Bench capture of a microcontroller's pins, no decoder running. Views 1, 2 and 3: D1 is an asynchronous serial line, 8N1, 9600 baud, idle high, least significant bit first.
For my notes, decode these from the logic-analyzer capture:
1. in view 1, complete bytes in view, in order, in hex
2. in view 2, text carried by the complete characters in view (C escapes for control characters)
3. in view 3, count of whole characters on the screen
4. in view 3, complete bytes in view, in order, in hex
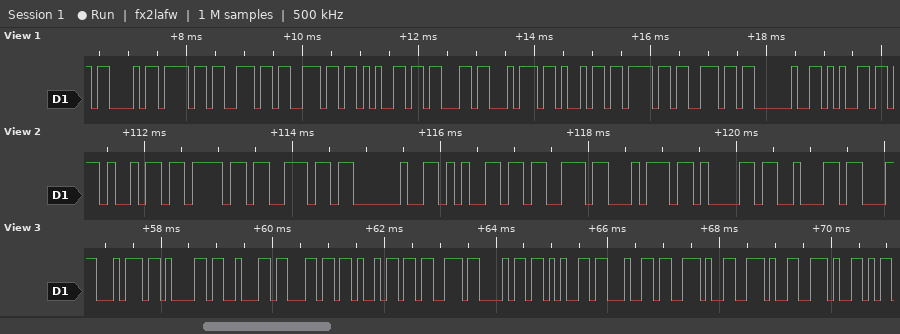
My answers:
43 6F 6E 6E 65 63 74 69 6F 6E 20 65
"ion estab"
12
74 61 62 6C 69 73 68 65 64 2E 2E 2E
